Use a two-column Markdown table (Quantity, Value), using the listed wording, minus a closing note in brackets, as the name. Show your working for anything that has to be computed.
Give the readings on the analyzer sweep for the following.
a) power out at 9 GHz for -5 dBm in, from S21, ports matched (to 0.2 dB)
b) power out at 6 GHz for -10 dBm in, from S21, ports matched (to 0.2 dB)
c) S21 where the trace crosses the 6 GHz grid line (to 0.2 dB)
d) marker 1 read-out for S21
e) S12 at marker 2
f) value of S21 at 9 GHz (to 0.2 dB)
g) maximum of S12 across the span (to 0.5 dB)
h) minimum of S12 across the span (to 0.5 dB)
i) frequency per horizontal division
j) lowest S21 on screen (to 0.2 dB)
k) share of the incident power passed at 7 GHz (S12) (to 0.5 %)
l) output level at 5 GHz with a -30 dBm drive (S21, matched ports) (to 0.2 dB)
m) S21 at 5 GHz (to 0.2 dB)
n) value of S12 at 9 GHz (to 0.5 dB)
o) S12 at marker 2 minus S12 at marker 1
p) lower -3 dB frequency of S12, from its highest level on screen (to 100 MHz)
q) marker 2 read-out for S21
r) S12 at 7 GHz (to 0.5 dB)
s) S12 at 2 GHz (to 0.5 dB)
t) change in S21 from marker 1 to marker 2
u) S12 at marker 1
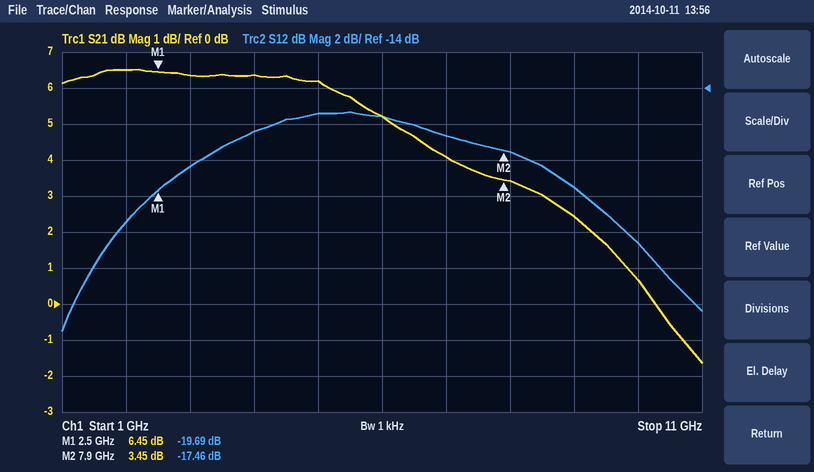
| Quantity | Value |
|---|---|
| power out at 9 GHz for -5 dBm in, from S21, ports matched | -5 dBm + (2.4 dB) = -2.6 dBm |
| power out at 6 GHz for -10 dBm in, from S21, ports matched | -10 dBm + (5.2 dB) = -4.8 dBm |
| S21 where the trace crosses the 6 GHz grid line | 5.2 dB |
| marker 1 read-out for S21 | 6.45 dB |
| S12 at marker 2 | -17.46 dB |
| value of S21 at 9 GHz | 2.4 dB |
| maximum of S12 across the span | -15.5 dB |
| minimum of S12 across the span | -27.5 dB |
| frequency per horizontal division | 1 GHz |
| lowest S21 on screen | -1.6 dB |
| share of the incident power passed at 7 GHz (S12) | 10^(-16.5/10) ≈ 2.24 %, so 2.0 % to the nearest 0.5 % |
| output level at 5 GHz with a -30 dBm drive (S21, matched ports) | -30 dBm + (6.2 dB) = -23.8 dBm |
| S21 at 5 GHz | 6.2 dB |
| value of S12 at 9 GHz | -19.5 dB |
| S12 at marker 2 minus S12 at marker 1 | -17.46 − (-19.69) = 2.23 dB |
| lower -3 dB frequency of S12, from its highest level on screen | 3.0 GHz |
| marker 2 read-out for S21 | 3.45 dB |
| S12 at 7 GHz | -16.5 dB |
| S12 at 2 GHz | -21.5 dB |
| change in S21 from marker 1 to marker 2 | 3.45 − (6.45) = -3.00 dB |
| S12 at marker 1 | -19.69 dB |
